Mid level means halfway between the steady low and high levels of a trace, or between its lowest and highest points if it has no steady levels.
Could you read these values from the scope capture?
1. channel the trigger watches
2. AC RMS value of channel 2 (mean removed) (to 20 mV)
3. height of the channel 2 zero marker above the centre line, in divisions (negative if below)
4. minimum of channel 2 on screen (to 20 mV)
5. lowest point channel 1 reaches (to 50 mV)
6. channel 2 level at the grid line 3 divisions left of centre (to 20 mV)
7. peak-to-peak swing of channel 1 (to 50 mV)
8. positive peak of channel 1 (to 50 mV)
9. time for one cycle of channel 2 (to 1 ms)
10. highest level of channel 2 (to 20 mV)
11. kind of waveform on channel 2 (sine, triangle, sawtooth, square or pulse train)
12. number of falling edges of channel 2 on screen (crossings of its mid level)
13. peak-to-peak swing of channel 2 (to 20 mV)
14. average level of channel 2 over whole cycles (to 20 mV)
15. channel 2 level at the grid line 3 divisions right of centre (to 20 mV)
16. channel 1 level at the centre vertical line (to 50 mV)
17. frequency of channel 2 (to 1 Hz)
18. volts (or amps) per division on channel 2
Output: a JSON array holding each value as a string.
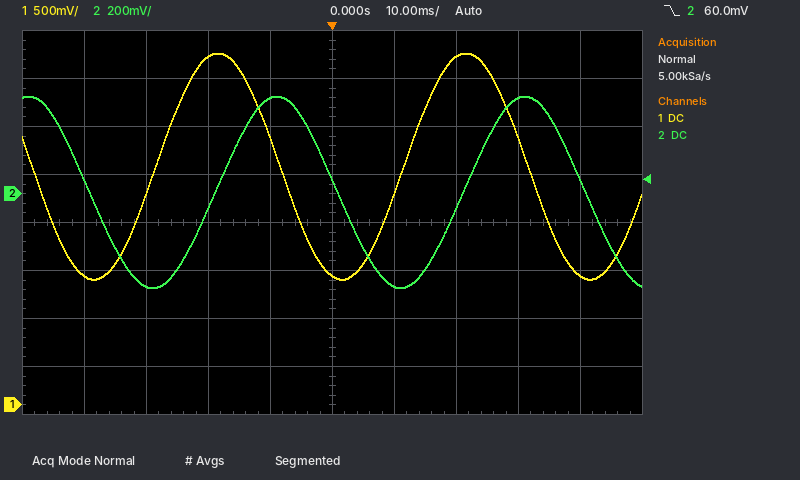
["channel 2", "280 mV", "+0.6 div", "-400 mV", "1.30 V", "-380 mV", "2.35 V", "3.65 V", "40 ms", "400 mV", "sine", "3", "800 mV", "0 mV", "400 mV", "1.35 V", "25 Hz", "200 mV"]
